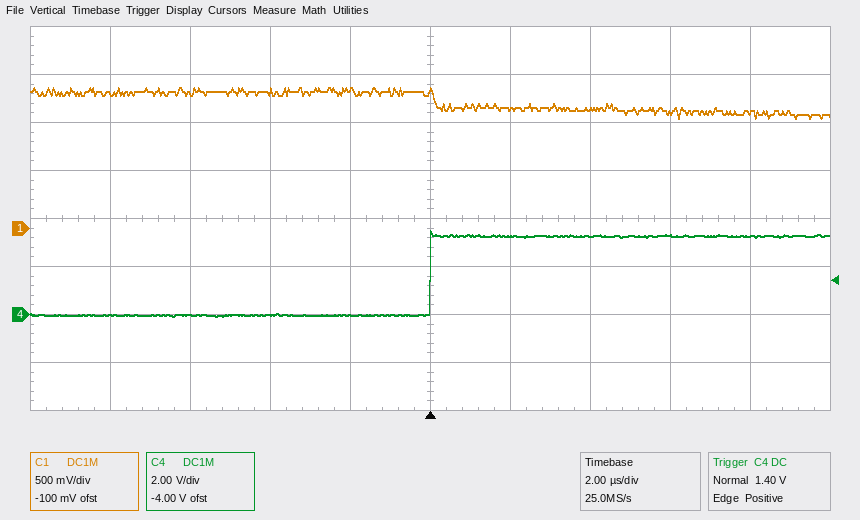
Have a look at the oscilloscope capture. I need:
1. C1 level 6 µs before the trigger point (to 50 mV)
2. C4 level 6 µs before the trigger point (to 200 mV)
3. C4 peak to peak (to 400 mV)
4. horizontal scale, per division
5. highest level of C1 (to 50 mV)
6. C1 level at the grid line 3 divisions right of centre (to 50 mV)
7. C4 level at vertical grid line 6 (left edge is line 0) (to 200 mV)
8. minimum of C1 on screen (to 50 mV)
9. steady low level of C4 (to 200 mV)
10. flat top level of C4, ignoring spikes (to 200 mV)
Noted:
1.40 V
0.0 V
3.6 V
2 µs
1.45 V
1.20 V
3.2 V
1.15 V
0.0 V
3.2 V
